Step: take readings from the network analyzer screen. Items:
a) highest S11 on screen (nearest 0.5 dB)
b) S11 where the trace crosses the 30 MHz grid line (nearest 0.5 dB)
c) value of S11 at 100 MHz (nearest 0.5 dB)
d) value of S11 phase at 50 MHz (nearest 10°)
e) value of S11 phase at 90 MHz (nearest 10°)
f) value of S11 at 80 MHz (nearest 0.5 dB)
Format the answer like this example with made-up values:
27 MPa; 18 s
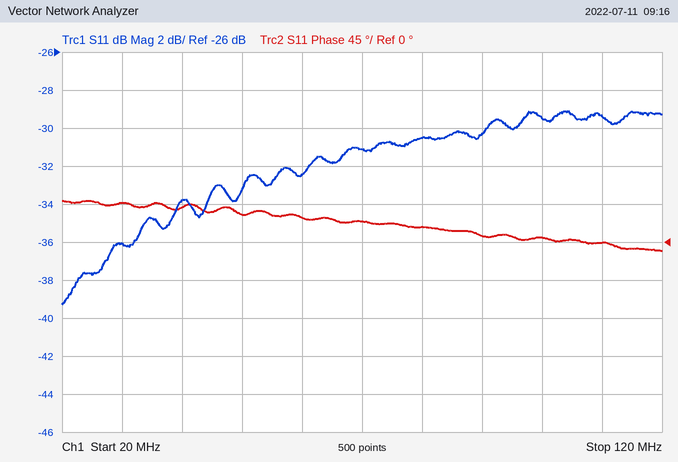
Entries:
-29.0 dB; -36.0 dB; -29.5 dB; 30°; 10°; -30.5 dB
